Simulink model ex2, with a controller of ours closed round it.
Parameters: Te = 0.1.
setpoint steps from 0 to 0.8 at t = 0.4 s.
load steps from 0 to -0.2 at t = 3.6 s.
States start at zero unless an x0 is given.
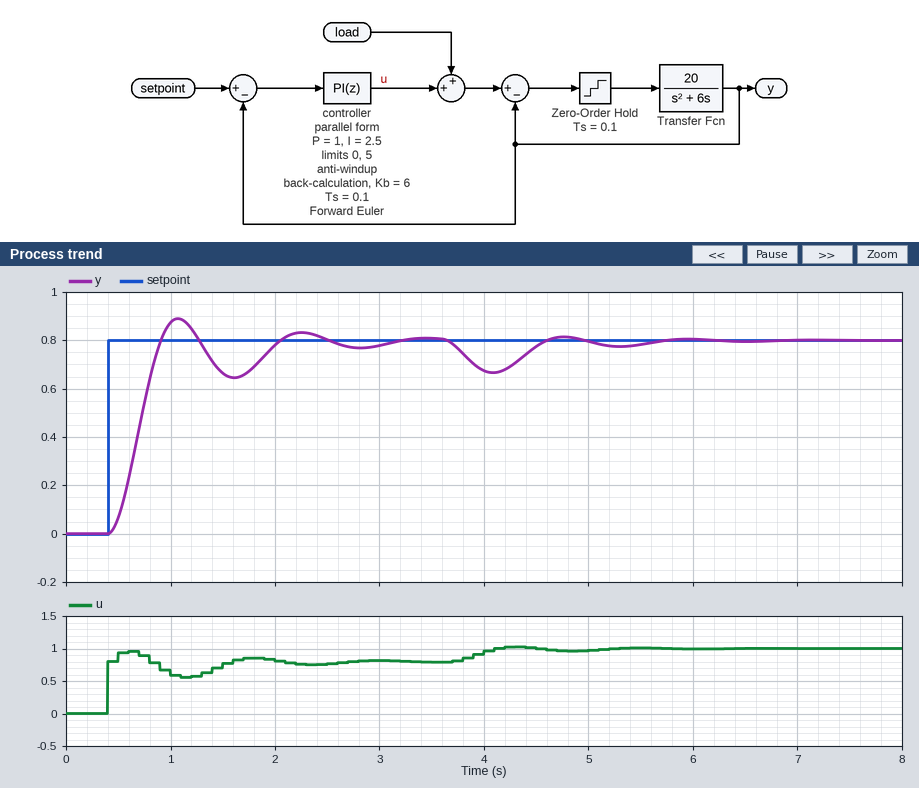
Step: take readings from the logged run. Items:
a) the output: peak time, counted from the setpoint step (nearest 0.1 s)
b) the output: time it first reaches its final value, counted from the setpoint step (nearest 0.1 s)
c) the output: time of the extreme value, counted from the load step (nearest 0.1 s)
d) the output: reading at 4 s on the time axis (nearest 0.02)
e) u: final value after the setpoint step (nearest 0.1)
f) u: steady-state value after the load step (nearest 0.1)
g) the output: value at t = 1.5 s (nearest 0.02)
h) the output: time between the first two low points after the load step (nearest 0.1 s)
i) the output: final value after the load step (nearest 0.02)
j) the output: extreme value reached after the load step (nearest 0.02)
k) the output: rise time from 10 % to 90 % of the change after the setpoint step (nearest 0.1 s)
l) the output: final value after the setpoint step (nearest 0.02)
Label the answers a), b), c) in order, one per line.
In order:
a) 0.7 s
b) 0.5 s
c) 0.5 s
d) 0.68
e) 0.8
f) 1.0
g) 0.66
h) 1.2 s
i) 0.80
j) 0.66
k) 0.3 s
l) 0.80
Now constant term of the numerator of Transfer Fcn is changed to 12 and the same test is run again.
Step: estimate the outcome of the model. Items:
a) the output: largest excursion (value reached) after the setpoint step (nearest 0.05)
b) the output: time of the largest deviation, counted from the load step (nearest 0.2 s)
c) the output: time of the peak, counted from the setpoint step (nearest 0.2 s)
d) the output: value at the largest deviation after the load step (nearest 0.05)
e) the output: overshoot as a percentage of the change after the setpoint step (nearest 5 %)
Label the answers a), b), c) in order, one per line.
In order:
a) 0.90
b) 0.6 s
c) 1.0 s
d) 0.70
e) 15 %
